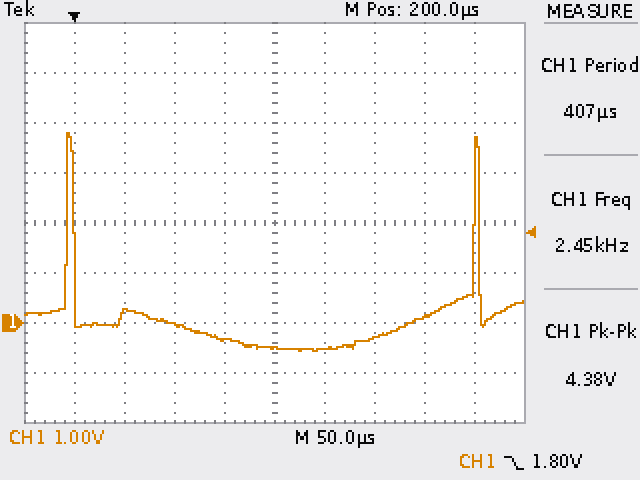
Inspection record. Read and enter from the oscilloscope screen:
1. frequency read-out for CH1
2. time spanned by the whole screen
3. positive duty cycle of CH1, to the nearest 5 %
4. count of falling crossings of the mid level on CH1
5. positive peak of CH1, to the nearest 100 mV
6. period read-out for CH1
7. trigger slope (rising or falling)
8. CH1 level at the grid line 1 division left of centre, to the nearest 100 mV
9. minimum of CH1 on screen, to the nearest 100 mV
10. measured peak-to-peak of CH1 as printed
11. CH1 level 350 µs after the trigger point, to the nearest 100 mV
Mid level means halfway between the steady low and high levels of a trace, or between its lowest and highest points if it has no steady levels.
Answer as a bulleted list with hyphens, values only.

- 2.45 kHz
- 500 µs
- 0 %
- 2
- 3.8 V
- 407 µs
- falling
- -300 mV
- -600 mV
- 4.38 V
- 100 mV
